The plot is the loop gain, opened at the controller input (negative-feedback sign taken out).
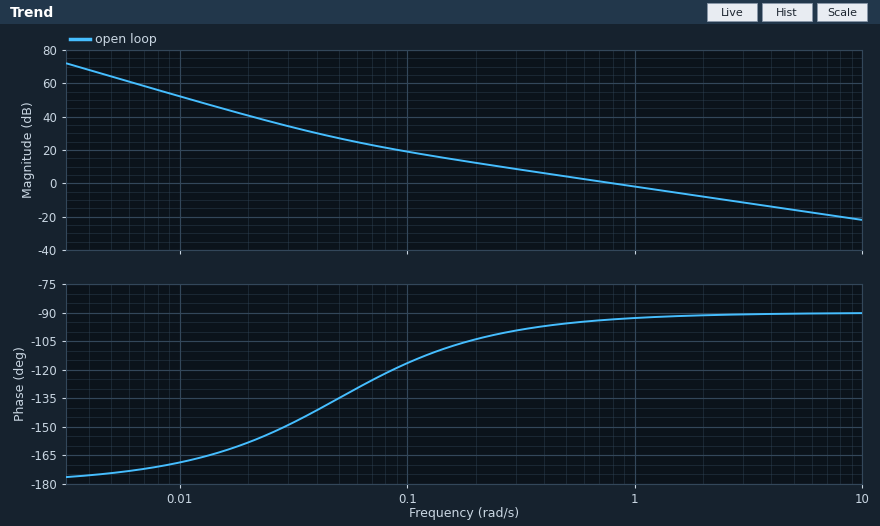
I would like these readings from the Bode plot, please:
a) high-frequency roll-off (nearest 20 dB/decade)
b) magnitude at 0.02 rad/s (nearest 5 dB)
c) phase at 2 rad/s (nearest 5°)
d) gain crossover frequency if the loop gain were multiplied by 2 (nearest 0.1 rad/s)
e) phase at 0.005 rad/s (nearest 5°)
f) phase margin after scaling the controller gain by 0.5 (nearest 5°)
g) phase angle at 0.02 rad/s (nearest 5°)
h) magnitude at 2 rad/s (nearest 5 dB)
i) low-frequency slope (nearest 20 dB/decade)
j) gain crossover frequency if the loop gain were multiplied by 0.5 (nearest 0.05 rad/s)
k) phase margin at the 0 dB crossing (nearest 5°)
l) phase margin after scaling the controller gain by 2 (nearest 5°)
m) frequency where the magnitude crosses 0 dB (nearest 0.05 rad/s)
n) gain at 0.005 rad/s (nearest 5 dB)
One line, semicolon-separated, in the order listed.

-20 dB/decade; 40 dB; -90°; 1.6 rad/s; -175°; 85°; -160°; -10 dB; -40 dB/decade; 0.40 rad/s; 85°; 90°; 0.80 rad/s; 65 dB
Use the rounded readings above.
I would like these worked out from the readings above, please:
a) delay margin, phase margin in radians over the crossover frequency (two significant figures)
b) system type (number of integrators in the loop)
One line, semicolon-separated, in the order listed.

1.9 s; 2
